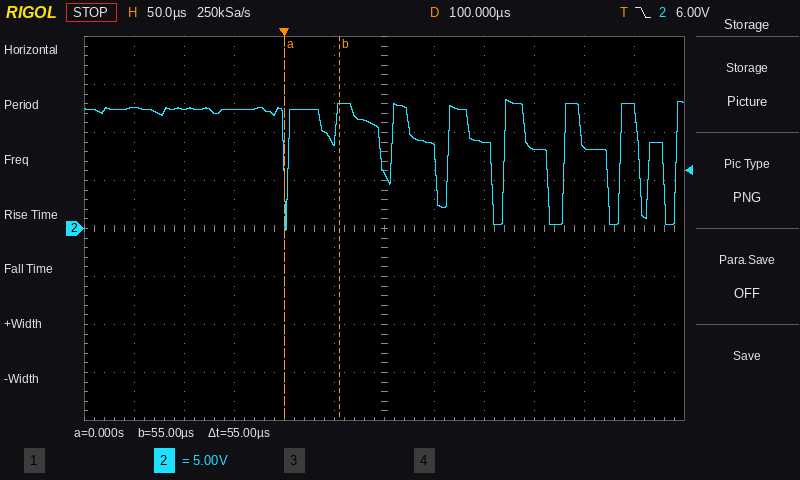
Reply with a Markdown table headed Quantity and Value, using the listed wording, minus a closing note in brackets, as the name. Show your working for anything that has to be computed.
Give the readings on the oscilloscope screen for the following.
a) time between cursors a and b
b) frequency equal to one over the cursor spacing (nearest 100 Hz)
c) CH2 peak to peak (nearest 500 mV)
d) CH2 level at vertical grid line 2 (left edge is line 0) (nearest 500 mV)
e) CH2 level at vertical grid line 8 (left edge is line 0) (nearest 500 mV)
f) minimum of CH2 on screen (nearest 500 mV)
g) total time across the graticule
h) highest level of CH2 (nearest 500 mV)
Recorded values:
| Quantity | Value |
|---|---|
| time between cursors a and b | 55 µs |
| frequency equal to one over the cursor spacing | 1 / 55 µs ≈ 18.2 kHz |
| CH2 peak to peak | 13.5 V − (0.0 V) = 13.5 V |
| CH2 level at vertical grid line 2 (left edge is line 0) | 12.5 V |
| CH2 level at vertical grid line 8 (left edge is line 0) | 9.0 V |
| minimum of CH2 on screen | 0.0 V |
| total time across the graticule | 600 µs |
| highest level of CH2 | 13.5 V |
